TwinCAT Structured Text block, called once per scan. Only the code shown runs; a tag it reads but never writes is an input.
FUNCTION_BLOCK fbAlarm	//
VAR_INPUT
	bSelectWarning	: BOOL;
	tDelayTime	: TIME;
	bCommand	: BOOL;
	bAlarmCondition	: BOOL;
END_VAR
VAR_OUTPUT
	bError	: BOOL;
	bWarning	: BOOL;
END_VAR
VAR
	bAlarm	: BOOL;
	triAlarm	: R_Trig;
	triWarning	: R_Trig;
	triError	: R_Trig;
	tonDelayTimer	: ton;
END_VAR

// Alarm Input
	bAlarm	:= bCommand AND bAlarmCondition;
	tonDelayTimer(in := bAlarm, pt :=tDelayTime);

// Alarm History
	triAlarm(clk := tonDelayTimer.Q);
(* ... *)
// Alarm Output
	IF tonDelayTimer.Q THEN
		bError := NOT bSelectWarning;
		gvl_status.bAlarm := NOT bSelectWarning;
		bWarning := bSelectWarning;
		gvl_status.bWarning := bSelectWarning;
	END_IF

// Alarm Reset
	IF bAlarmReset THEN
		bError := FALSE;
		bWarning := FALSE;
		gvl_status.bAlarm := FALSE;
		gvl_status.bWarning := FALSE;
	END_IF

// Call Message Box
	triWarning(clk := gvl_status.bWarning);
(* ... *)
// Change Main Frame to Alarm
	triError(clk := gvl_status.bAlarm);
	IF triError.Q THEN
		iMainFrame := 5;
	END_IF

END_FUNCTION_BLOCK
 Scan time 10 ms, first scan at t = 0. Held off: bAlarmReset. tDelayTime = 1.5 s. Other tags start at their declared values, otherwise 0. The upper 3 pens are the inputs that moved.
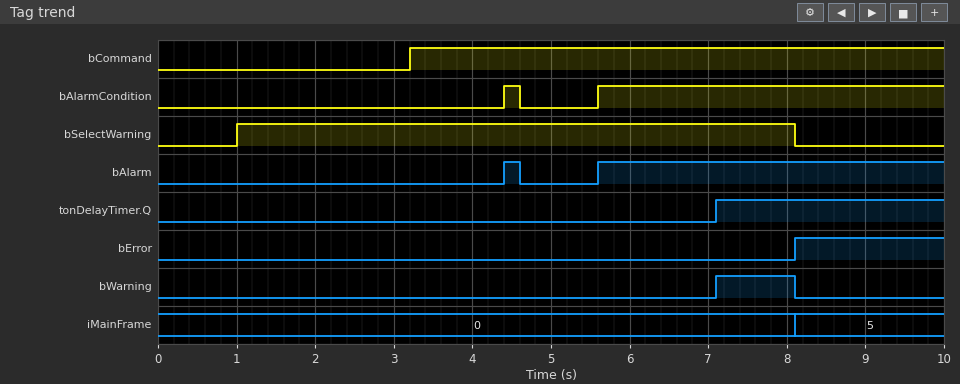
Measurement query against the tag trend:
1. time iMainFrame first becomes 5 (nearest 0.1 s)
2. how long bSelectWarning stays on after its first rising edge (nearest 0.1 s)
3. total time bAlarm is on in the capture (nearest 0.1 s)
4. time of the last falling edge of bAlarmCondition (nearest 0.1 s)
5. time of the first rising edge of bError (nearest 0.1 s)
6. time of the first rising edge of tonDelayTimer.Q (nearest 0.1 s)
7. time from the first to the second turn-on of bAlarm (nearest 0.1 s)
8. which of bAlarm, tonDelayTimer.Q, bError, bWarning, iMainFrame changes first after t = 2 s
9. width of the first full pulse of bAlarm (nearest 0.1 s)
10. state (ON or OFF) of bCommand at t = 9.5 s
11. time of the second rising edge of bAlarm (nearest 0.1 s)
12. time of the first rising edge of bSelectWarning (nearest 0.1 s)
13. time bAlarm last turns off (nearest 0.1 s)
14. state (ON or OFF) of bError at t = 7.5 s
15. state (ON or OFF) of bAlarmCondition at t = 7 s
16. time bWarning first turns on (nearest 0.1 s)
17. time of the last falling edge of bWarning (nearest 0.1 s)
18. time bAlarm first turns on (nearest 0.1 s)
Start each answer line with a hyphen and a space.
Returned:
- 8.1 s
- 7.1 s
- 4.6 s
- 4.6 s
- 8.1 s
- 7.1 s
- 1.2 s
- bAlarm
- 0.2 s
- ON
- 5.6 s
- 1.0 s
- 4.6 s
- OFF
- ON
- 7.1 s
- 8.1 s
- 4.4 s
